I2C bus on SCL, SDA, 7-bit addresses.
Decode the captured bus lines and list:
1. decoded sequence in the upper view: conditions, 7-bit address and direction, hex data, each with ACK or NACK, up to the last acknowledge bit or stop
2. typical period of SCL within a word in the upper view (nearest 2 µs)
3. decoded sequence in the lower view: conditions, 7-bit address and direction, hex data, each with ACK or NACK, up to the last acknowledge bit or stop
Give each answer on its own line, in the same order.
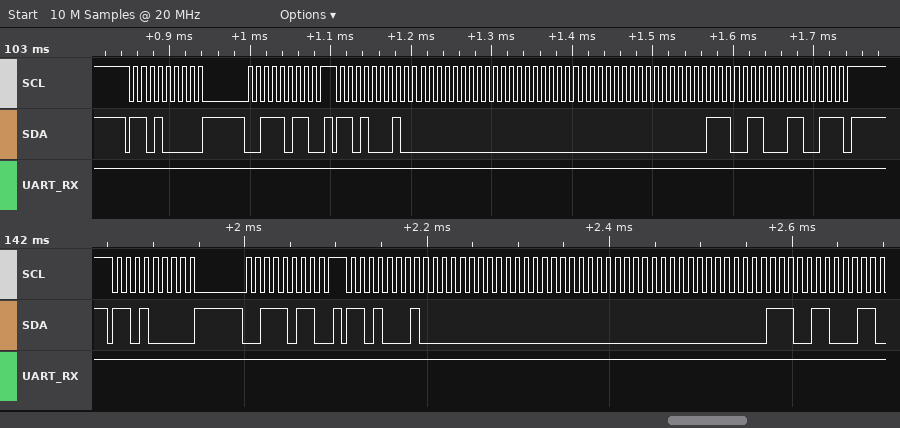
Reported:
start, address 68 write ACK, 3B ACK, stop, start, address 68 read ACK, 00 ACK, 00 ACK, 00 ACK, 00 ACK, 73 ACK, 33 NACK, stop
10 µs
start, address 68 write ACK, 3B ACK, stop, start, address 68 read ACK, 00 ACK, 00 ACK, 00 ACK, 00 ACK, 73 ACK
